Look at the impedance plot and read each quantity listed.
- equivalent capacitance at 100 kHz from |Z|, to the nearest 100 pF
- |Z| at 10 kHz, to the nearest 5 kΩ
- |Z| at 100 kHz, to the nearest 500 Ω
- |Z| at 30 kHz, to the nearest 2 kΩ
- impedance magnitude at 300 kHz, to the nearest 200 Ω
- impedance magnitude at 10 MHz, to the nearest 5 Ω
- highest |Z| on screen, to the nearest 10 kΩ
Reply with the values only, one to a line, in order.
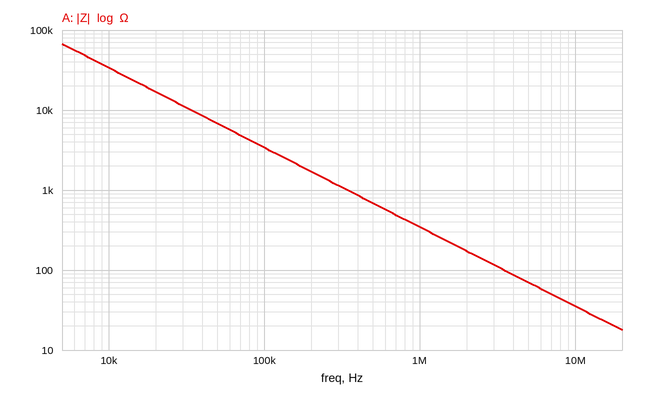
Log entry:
500 pF
35 kΩ
3.5 kΩ
12 kΩ
1.2 kΩ
35 Ω
70 kΩ
